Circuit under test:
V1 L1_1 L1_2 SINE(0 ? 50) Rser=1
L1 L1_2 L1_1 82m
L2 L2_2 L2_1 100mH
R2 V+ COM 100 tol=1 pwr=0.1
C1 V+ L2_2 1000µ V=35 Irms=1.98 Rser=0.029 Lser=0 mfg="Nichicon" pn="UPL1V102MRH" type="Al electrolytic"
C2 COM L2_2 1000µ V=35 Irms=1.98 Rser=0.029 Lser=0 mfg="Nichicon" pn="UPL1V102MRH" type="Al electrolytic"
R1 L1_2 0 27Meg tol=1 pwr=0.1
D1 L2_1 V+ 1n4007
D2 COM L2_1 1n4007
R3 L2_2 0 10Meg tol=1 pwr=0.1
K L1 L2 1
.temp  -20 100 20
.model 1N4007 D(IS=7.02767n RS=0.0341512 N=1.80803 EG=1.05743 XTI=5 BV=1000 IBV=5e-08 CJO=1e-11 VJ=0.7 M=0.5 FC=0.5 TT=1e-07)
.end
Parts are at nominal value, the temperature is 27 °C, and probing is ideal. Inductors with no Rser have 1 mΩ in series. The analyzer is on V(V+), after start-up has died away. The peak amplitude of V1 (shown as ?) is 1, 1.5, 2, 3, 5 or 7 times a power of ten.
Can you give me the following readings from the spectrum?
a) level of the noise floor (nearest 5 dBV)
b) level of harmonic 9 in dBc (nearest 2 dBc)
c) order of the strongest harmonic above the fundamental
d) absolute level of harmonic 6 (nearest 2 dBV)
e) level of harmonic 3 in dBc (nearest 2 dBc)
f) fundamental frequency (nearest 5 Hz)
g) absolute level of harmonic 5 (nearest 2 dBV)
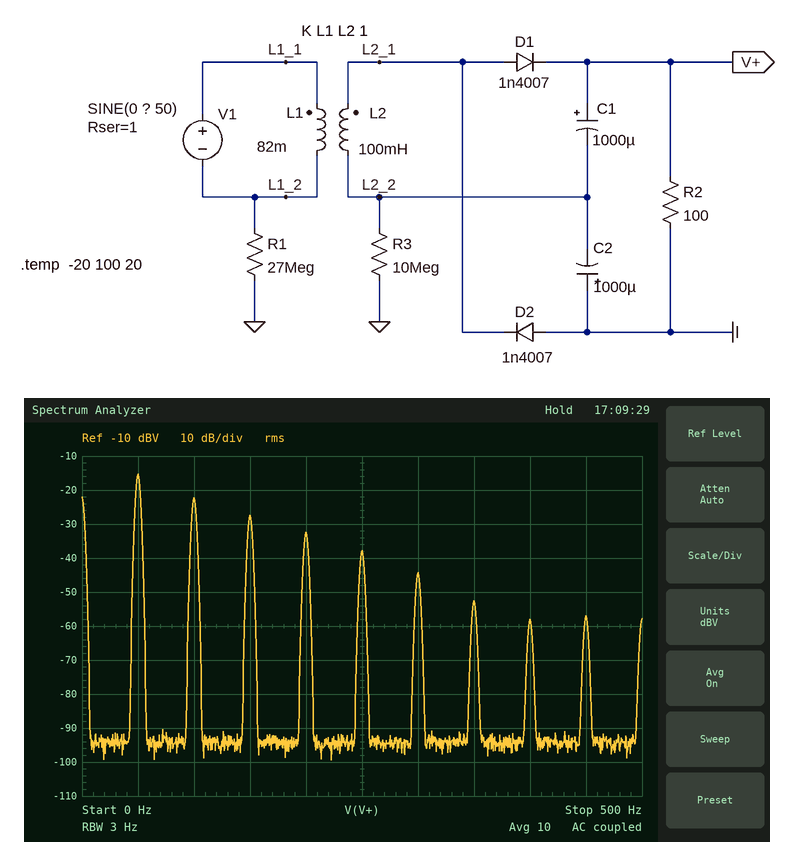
-95 dBV
-42 dBc
2
-44 dBV
-12 dBc
50 Hz
-38 dBV
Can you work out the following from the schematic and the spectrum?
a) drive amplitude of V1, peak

3 V
